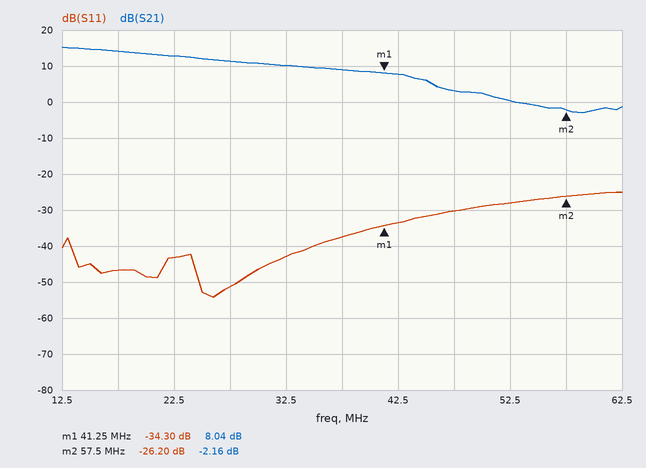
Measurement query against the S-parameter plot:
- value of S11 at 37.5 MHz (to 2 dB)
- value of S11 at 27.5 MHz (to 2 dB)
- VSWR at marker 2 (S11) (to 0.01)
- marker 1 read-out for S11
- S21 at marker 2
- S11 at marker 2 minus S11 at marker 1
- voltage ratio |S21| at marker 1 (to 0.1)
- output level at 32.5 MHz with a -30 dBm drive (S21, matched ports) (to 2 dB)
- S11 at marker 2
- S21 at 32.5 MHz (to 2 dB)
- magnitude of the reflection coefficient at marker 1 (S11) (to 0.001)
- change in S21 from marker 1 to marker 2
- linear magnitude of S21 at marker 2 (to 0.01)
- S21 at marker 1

-38 dB
-52 dB
1.10
-34.30 dB
-2.16 dB
8.10 dB
2.5
-20 dBm
-26.20 dB
10 dB
0.019
-10.20 dB
0.78
8.04 dB
